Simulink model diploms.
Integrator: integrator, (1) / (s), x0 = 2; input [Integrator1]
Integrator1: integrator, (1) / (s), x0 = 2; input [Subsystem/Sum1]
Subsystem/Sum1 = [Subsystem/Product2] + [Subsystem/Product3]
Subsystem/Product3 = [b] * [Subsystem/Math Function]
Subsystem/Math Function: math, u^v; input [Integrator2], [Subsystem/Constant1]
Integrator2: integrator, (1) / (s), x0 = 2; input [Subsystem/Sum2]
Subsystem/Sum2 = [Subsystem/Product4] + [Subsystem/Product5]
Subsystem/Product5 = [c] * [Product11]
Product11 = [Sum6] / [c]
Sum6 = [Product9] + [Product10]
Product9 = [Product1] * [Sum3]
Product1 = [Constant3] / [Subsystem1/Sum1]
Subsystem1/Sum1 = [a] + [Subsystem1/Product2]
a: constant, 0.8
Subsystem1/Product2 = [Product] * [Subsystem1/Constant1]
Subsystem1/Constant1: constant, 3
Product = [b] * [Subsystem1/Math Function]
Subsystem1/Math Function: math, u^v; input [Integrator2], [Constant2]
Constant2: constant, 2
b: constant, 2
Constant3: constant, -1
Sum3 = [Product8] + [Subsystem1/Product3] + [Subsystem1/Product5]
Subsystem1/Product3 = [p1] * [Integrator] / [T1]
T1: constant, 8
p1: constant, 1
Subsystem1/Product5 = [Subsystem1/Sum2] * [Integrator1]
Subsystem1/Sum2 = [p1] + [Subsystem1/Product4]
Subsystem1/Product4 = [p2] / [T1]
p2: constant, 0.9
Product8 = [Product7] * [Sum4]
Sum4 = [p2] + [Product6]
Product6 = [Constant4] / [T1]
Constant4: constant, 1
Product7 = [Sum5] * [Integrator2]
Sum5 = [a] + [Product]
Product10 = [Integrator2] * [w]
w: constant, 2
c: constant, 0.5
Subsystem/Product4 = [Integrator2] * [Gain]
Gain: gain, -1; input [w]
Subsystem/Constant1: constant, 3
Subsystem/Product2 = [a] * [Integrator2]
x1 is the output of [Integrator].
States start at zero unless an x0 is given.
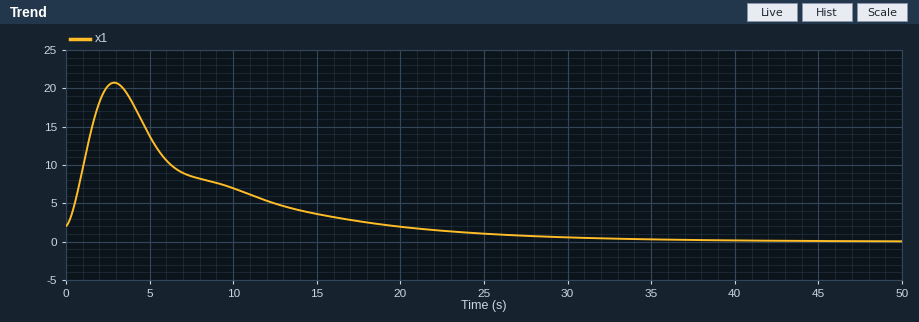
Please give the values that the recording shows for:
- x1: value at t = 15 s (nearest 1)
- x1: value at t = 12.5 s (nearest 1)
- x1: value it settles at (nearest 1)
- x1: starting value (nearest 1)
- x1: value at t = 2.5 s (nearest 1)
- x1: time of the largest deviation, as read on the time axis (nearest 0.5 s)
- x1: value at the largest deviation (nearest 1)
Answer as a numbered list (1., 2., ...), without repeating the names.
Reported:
1. 4
2. 5
3. 0
4. 2
5. 20
6. 3.0 s
7. 21
